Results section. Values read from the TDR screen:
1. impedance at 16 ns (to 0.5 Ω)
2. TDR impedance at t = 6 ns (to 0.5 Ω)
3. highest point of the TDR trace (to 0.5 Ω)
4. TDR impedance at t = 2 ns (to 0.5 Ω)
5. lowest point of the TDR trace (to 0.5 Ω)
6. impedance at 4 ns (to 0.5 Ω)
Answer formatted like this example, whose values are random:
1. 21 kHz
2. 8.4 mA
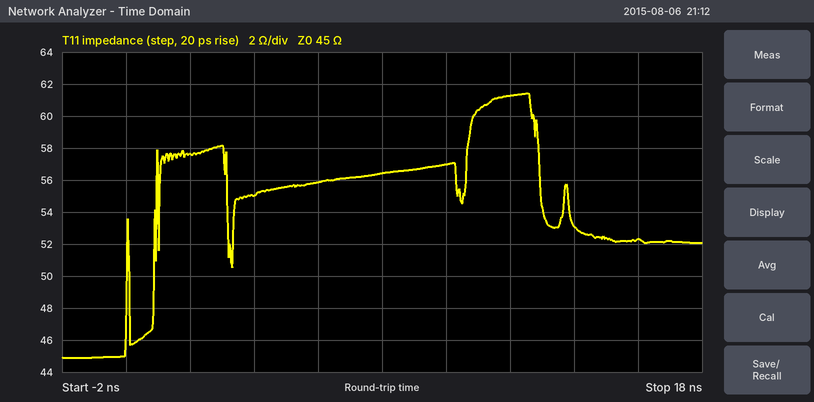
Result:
1. 52.5 Ω
2. 56.0 Ω
3. 61.5 Ω
4. 57.5 Ω
5. 45.0 Ω
6. 55.0 Ω
